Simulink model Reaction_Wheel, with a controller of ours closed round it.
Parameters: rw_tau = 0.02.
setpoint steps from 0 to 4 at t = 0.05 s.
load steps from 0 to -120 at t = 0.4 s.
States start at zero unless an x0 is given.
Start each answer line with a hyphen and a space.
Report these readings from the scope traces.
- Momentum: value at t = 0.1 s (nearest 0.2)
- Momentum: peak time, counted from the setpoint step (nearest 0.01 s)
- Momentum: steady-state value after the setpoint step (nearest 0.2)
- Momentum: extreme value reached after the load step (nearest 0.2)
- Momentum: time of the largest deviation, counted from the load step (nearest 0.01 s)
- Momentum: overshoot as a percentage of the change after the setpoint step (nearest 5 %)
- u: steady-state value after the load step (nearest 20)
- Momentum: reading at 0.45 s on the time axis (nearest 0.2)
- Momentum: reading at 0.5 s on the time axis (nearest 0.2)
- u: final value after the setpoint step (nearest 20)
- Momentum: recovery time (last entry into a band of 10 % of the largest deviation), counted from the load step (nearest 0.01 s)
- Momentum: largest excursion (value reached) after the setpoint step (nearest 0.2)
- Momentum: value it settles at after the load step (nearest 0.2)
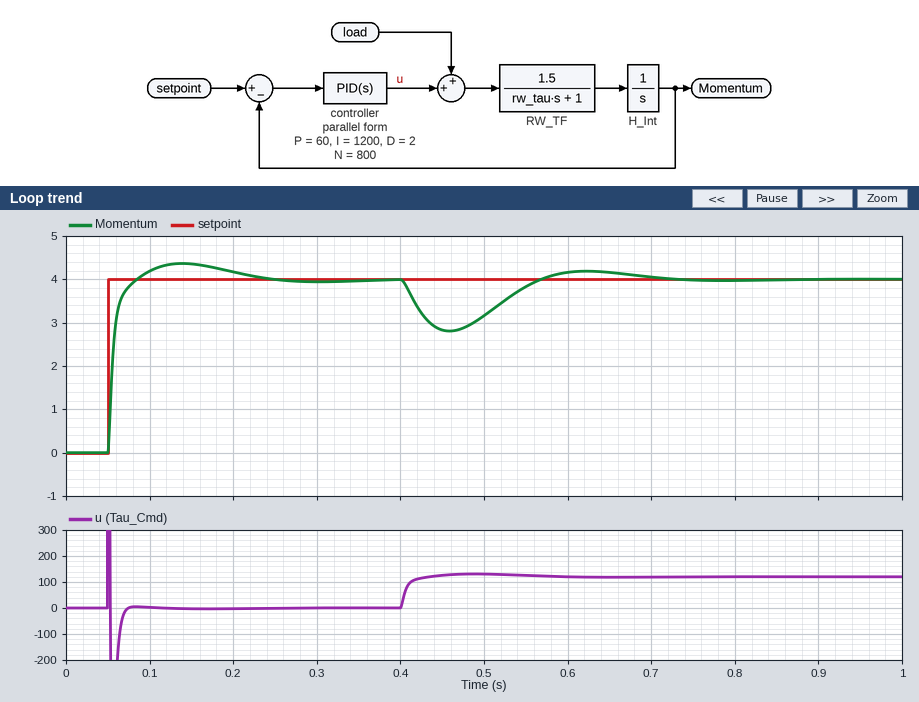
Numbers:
- 4.2
- 0.09 s
- 4.0
- 2.8
- 0.06 s
- 10 %
- 120
- 2.8
- 3.2
- 0
- 0.27 s
- 4.4
- 4.0
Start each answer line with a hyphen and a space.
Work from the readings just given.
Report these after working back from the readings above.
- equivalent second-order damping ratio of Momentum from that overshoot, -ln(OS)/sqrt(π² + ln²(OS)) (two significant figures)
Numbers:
- 0.59
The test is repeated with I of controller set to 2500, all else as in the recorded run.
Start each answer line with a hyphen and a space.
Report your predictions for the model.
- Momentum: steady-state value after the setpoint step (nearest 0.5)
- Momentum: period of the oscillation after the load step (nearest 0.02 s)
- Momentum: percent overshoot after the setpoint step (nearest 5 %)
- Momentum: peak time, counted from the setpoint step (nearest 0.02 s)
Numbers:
- 4.0
- 0.20 s
- 15 %
- 0.06 s
